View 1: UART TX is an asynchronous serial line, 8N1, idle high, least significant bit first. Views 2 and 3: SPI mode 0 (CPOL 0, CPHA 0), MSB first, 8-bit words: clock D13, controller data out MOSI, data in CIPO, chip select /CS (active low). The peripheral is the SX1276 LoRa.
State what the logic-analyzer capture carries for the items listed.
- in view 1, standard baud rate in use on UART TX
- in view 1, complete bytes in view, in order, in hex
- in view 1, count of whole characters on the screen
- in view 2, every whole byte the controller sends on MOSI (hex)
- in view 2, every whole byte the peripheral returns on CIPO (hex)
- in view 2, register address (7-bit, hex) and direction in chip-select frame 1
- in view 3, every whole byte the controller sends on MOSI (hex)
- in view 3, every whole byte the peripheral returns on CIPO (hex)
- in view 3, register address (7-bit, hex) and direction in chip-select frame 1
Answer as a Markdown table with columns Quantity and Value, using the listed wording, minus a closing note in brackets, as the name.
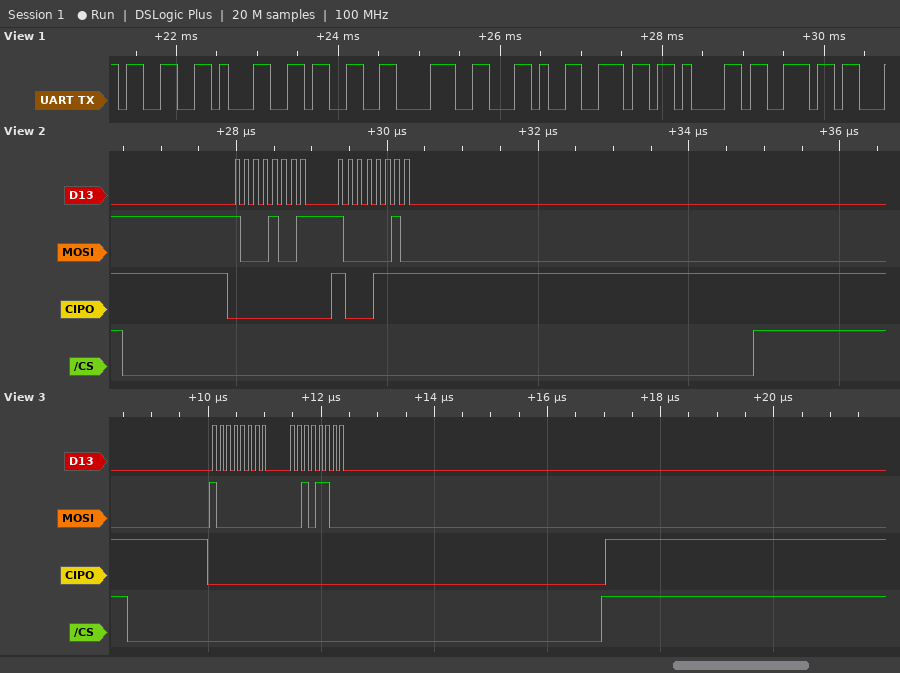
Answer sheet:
| Quantity | Value |
|---|---|
| in view 1, standard baud rate in use on UART TX | 9600 baud |
| in view 1, complete bytes in view, in order, in hex | 33 31 33 38 2C 6E 61 6E |
| in view 1, count of whole characters on the screen | 8 |
| in view 2, every whole byte the controller sends on MOSI | 89 82 |
| in view 2, every whole byte the peripheral returns on CIPO | 00 8F |
| in view 2, register address (7-bit, hex) and direction in chip-select frame 1 | 0x09 write |
| in view 3, every whole byte the controller sends on MOSI | 0x80 0x2C |
| in view 3, every whole byte the peripheral returns on CIPO | 0x00 0x00 |
| in view 3, register address (7-bit, hex) and direction in chip-select frame 1 | 0x00 write |
